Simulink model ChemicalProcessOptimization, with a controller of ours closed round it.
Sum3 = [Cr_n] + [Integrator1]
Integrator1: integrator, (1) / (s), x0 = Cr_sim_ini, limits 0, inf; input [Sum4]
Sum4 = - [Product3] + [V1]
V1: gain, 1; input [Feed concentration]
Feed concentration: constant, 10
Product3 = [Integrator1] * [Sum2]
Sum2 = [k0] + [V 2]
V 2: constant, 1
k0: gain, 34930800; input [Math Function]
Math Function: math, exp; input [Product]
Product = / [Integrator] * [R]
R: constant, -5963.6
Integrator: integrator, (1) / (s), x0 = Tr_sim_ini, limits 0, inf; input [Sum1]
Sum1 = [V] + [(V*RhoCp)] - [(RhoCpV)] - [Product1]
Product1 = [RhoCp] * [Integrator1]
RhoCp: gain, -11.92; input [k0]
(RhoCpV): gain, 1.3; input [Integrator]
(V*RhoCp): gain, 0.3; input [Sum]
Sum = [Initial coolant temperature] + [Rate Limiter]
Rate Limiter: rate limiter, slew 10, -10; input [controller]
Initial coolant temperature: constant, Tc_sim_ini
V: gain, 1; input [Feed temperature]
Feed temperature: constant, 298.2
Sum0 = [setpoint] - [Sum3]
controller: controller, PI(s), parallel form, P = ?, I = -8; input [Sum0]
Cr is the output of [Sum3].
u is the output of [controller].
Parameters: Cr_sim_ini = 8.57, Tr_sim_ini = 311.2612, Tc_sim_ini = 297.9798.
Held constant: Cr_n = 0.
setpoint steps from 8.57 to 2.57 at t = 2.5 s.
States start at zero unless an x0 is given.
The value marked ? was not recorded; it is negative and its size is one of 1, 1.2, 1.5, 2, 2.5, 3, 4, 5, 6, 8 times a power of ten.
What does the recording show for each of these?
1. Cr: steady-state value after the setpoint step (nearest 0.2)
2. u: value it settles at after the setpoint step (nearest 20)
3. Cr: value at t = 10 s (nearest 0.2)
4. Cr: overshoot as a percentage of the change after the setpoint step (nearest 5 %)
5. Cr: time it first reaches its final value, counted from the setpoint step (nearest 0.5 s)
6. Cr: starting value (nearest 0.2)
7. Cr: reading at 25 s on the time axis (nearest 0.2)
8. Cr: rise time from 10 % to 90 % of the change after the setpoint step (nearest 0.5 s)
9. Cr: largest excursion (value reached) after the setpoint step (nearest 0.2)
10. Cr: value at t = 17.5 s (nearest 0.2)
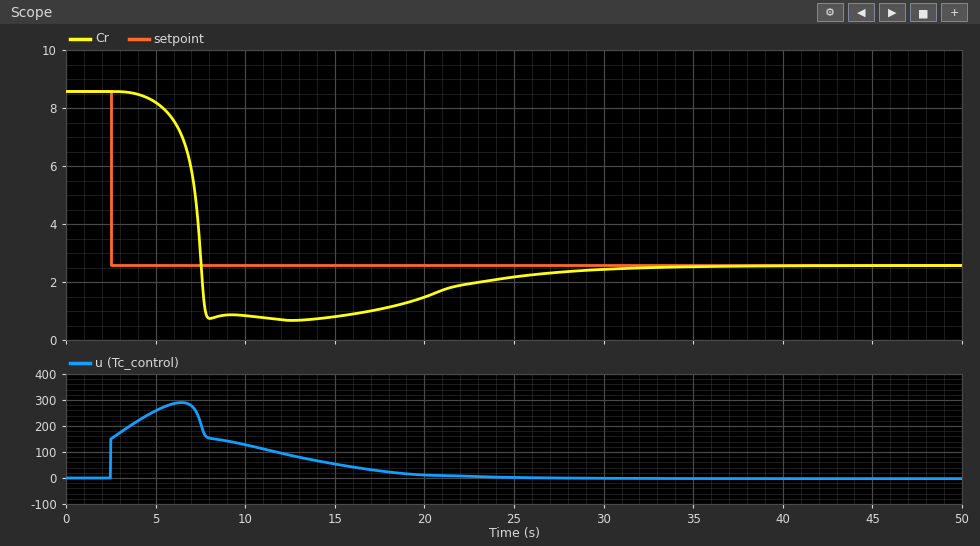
2.6
0
0.8
30 %
5.0 s
8.6
2.2
2.0 s
0.6
1.0
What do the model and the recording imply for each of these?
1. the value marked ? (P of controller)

-25
